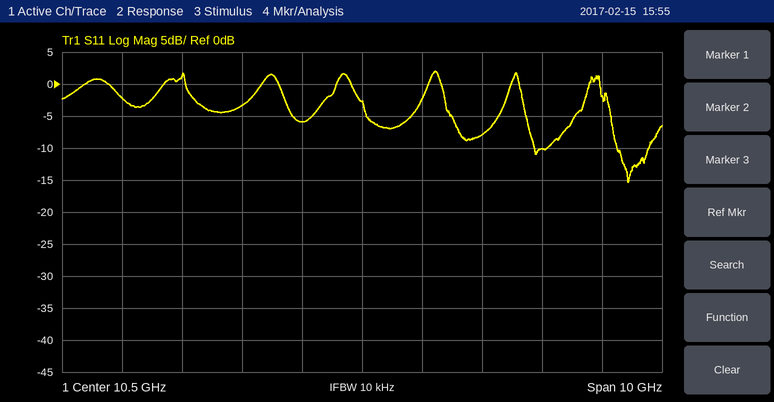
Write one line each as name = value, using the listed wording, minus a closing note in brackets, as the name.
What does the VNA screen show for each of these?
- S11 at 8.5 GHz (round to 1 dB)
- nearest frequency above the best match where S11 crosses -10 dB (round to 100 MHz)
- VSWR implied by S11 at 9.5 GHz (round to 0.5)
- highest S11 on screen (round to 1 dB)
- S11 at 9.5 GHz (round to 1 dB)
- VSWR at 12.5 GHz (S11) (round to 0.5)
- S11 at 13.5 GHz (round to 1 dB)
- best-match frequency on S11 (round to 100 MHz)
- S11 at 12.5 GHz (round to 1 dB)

S11 at 8.5 GHz = -3 dB
nearest frequency above the best match where S11 crosses -10 dB = 15.3 GHz
VSWR implied by S11 at 9.5 GHz = 3.0
highest S11 on screen = 2 dB
S11 at 9.5 GHz = -6 dB
VSWR at 12.5 GHz (S11) = 2.5
S11 at 13.5 GHz = -10 dB
best-match frequency on S11 = 14.9 GHz
S11 at 12.5 GHz = -8 dB
